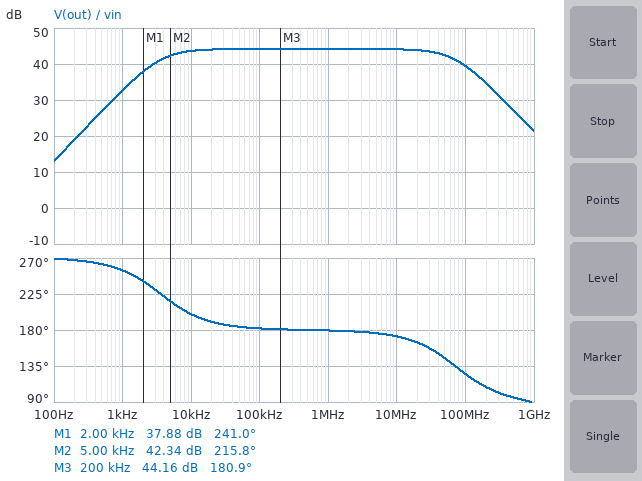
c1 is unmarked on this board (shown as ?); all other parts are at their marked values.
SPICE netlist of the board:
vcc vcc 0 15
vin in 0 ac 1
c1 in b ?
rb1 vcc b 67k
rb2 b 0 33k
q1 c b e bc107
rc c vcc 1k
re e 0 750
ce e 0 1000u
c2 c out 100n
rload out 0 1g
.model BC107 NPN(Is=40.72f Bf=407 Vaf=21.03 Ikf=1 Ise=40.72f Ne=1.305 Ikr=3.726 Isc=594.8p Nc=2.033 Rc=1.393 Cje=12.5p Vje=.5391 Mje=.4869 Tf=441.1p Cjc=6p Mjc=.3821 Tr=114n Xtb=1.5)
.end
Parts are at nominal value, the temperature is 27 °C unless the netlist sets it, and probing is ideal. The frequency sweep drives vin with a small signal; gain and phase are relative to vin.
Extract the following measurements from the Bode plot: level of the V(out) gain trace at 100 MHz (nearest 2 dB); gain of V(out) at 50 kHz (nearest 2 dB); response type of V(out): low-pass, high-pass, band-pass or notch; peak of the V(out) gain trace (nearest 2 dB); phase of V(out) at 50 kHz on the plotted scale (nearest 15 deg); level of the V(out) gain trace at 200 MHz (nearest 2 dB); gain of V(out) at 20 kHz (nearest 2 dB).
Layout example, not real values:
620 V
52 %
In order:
40 dB
44 dB
band-pass
44 dB
180 deg
34 dB
44 dB
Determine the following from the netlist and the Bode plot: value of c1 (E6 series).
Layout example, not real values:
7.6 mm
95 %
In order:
33 nF
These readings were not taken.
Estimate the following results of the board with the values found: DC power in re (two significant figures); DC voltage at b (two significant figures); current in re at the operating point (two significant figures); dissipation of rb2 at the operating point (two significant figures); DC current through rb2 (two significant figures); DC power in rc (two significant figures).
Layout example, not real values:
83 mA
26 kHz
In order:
20 mW
4.5 V
5.1 mA
610 µW
140 µA
26 mW
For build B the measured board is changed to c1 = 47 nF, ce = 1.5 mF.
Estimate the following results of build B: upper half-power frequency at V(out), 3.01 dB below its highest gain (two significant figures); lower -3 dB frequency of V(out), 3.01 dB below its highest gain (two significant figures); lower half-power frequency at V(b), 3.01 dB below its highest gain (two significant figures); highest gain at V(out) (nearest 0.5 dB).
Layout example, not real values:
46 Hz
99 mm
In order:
71 MHz
2.5 kHz
2.6 kHz
44.0 dB
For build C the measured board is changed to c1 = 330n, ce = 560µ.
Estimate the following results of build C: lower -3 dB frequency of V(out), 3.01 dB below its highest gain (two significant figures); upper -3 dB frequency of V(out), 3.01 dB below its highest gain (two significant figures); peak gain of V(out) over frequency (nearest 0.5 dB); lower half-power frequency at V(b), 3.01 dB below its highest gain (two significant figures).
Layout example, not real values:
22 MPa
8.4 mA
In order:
410 Hz
71 MHz
44.5 dB
400 Hz
